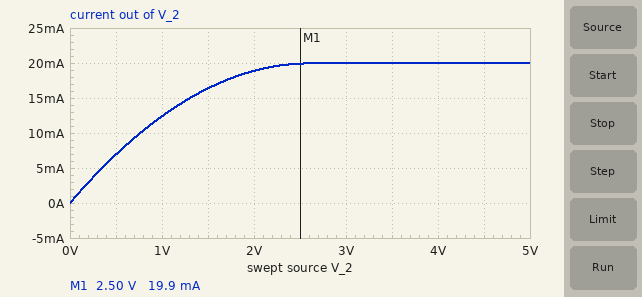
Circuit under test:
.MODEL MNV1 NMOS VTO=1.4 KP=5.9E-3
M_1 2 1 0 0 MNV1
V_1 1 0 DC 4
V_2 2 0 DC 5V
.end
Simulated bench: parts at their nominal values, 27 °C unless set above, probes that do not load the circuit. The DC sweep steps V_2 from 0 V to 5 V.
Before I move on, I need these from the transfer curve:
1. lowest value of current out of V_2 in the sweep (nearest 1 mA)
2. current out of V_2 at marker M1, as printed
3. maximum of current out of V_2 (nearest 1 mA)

0 A
19.9 mA
20 mA
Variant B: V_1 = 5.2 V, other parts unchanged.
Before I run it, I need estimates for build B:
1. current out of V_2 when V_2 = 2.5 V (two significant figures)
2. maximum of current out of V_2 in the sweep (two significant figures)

38 mA
43 mA
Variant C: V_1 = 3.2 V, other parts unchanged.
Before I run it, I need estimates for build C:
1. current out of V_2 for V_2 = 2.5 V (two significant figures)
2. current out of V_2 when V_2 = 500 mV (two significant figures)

9.6 mA
4.6 mA
